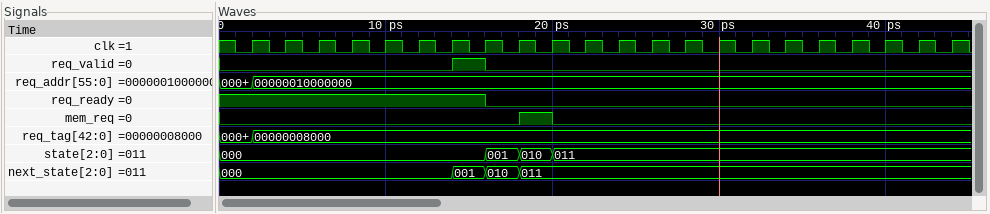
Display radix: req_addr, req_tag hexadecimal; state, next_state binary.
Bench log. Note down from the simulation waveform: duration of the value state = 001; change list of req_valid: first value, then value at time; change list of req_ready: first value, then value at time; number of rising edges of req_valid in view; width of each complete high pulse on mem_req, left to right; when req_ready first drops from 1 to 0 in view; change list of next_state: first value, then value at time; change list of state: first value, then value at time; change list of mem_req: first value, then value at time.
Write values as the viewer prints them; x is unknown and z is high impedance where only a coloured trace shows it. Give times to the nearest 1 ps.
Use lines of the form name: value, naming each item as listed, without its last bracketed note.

duration of the value state = 001: 2 ps
change list of req_valid: first value, then value at time: 0, 1 at 14 ps, 0 at 16 ps
change list of req_ready: first value, then value at time: 1, 0 at 16 ps
number of rising edges of req_valid in view: 1
width of each complete high pulse on mem_req, left to right: 2 ps
when req_ready first drops from 1 to 0 in view: 16 ps
change list of next_state: first value, then value at time: 000, 001 at 14 ps, 010 at 16 ps, 011 at 18 ps
change list of state: first value, then value at time: 000, 001 at 16 ps, 010 at 18 ps, 011 at 20 ps
change list of mem_req: first value, then value at time: 0, 1 at 18 ps, 0 at 20 ps
